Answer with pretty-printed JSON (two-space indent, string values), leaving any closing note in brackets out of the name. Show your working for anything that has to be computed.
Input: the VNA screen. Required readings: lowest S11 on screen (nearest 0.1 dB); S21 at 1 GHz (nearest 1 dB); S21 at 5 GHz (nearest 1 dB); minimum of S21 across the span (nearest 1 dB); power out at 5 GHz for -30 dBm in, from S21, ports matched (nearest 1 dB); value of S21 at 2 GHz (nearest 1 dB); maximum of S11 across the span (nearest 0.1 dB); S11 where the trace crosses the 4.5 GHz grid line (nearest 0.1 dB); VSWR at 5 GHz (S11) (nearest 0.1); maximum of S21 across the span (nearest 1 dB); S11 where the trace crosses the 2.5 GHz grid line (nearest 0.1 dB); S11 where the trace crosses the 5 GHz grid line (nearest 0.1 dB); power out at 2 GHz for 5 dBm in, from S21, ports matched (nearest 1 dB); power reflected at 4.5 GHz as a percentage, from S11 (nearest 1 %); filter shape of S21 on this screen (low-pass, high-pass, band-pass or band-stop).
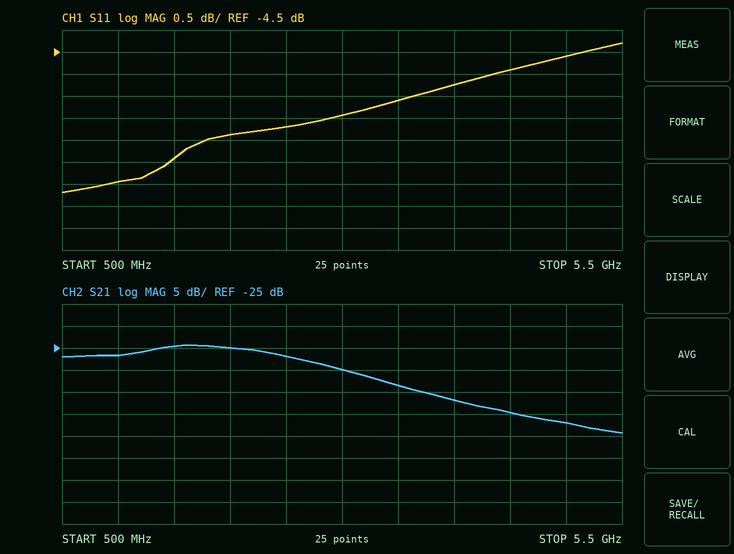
{
  "lowest S11 on screen": "-7.7 dB",
  "S21 at 1 GHz": "-27 dB",
  "S21 at 5 GHz": "-42 dB",
  "minimum of S21 across the span": "-44 dB",
  "power out at 5 GHz for -30 dBm in, from S21, ports matched": "-30 dBm + (-42 dB) = -72 dBm",
  "value of S21 at 2 GHz": "-25 dB",
  "maximum of S11 across the span": "-4.3 dB",
  "S11 where the trace crosses the 4.5 GHz grid line": "-4.9 dB",
  "VSWR at 5 GHz (S11)": "|Γ| = 10^(-4.6/20) = 0.5888; VSWR = (1 + 0.5888)/(1 − 0.5888) ≈ 3.9",
  "maximum of S21 across the span": "-24 dB",
  "S11 where the trace crosses the 2.5 GHz grid line": "-6.2 dB",
  "S11 where the trace crosses the 5 GHz grid line": "-4.6 dB",
  "power out at 2 GHz for 5 dBm in, from S21, ports matched": "5 dBm + (-25 dB) = -20 dBm",
  "power reflected at 4.5 GHz as a percentage, from S11": "10^(-4.9/10) ≈ 32 %",
  "filter shape of S21 on this screen": "low-pass"
}
